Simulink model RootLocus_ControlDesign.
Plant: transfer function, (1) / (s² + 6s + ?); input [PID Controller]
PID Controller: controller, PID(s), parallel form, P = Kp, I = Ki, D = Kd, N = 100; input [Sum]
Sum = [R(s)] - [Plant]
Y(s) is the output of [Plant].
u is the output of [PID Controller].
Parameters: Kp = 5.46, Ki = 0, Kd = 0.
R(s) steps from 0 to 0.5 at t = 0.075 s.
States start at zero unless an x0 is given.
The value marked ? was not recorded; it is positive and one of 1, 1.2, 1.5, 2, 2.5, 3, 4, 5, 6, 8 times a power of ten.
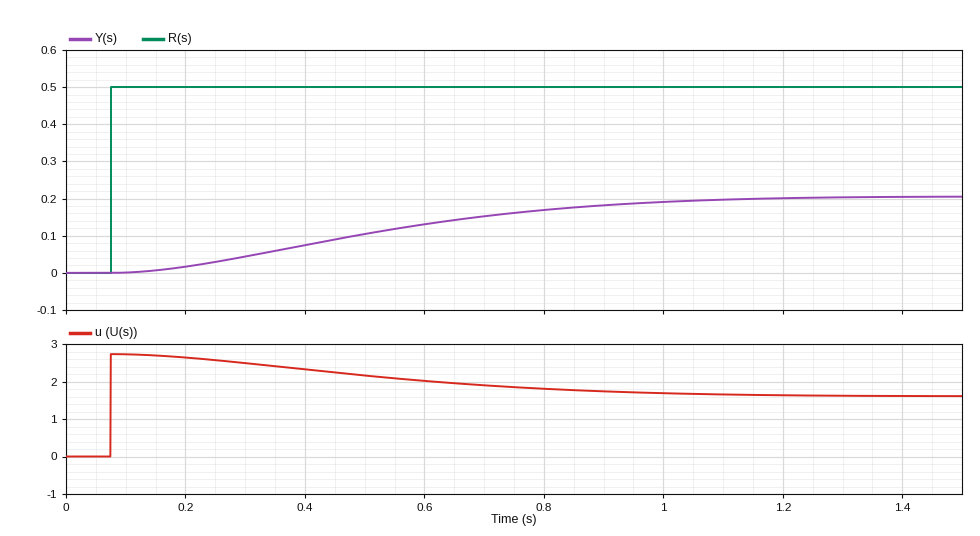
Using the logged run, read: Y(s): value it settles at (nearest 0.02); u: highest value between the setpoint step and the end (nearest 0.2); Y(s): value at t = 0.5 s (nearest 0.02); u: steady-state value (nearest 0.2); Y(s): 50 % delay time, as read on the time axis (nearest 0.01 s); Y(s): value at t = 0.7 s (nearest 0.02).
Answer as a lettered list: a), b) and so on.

a) 0.20
b) 2.8
c) 0.10
d) 1.6
e) 0.49 s
f) 0.16
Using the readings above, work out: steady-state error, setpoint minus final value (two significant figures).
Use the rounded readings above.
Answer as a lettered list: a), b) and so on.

a) 0.30
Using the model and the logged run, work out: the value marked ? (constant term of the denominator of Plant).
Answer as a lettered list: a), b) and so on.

a) 8
